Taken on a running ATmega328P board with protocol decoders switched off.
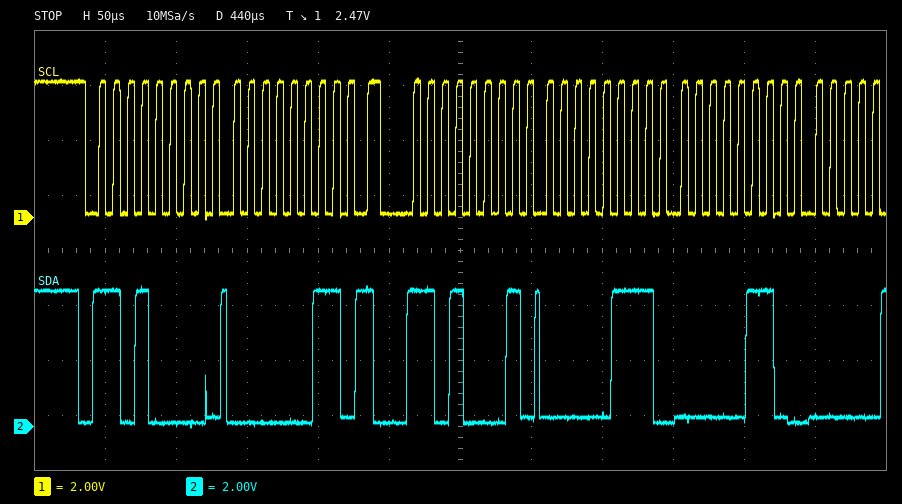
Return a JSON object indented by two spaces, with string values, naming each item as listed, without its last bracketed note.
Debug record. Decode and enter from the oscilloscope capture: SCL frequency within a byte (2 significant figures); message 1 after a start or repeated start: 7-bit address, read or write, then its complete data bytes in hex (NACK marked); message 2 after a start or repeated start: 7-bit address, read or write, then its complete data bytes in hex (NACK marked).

{
  "SCL frequency within a byte": "100 kHz",
  "message 1 after a start or repeated start: 7-bit address, read or write, then its complete data bytes in hex": "0x68 write: 03",
  "message 2 after a start or repeated start: 7-bit address, read or write, then its complete data bytes in hex": "0x68 read: 07 06"
}
